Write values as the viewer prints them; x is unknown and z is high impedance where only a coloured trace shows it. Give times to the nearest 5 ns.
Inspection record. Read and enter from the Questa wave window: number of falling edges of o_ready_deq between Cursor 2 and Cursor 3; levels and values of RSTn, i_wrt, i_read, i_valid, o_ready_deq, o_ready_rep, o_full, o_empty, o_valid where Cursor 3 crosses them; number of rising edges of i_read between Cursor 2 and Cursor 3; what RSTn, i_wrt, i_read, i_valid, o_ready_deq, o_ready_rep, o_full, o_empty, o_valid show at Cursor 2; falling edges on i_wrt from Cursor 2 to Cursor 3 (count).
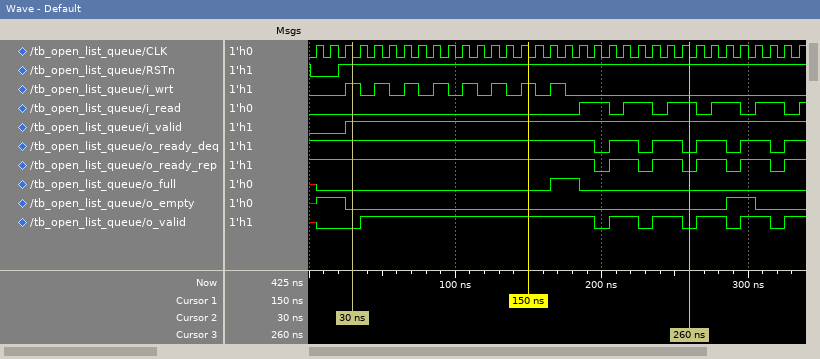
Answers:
3
RSTn=1, i_wrt=0, i_read=1, i_valid=1, o_ready_deq=0, o_ready_rep=0, o_full=0, o_empty=0, o_valid=0
3
RSTn=1, i_wrt=1, i_read=0, i_valid=1, o_ready_deq=1, o_ready_rep=1, o_full=0, o_empty=0, o_valid=0
8
